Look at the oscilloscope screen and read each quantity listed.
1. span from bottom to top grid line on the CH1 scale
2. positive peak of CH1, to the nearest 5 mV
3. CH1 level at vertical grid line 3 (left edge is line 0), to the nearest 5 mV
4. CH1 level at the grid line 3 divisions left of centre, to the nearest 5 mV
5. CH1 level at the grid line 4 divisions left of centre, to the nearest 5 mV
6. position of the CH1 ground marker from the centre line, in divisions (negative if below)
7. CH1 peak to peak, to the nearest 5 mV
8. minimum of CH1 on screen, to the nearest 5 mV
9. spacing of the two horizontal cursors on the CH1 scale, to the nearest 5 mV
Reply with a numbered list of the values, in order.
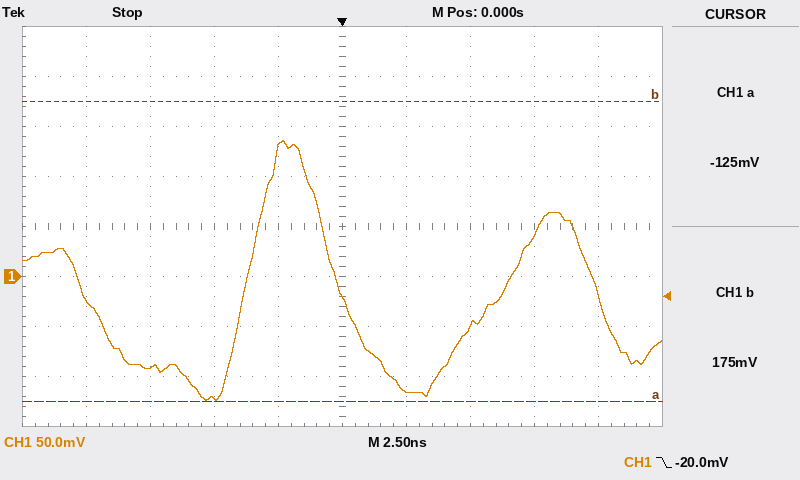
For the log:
1. 400 mV
2. 135 mV
3. -120 mV
4. -90 mV
5. -25 mV
6. -1.0 div
7. 260 mV
8. -125 mV
9. 300 mV
